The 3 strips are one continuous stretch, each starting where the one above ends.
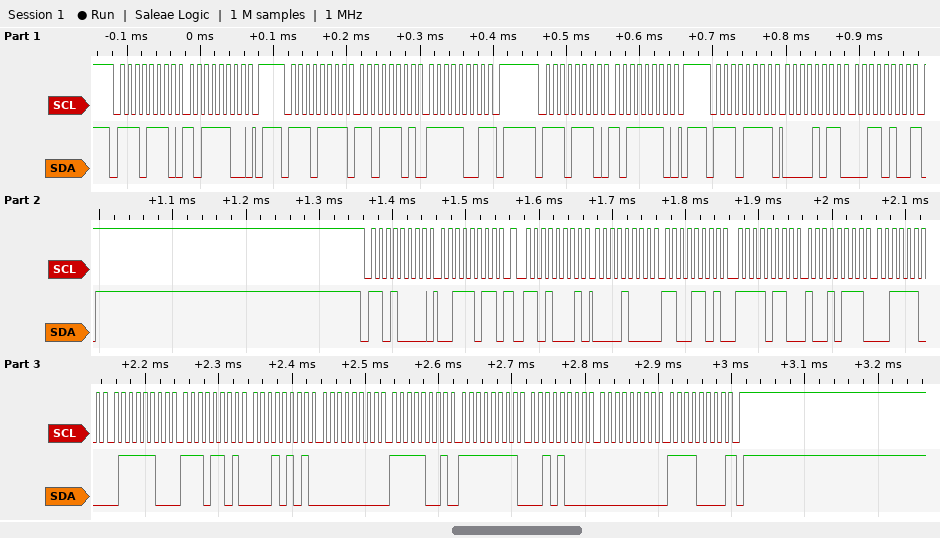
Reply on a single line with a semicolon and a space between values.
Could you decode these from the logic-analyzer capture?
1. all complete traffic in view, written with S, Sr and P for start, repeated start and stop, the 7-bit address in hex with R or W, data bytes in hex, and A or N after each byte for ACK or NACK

S 77W A BC A P S 77R A DD A F9 N P S 77W A BE A P S 77R A 0B A 34 N P S 68W A 3B A Sr 68R A 08 A CD A F6 A 97 A 3C A 7C A ED A 15 A 00 A F9 A FF A 28 A 00 A F0 N P
